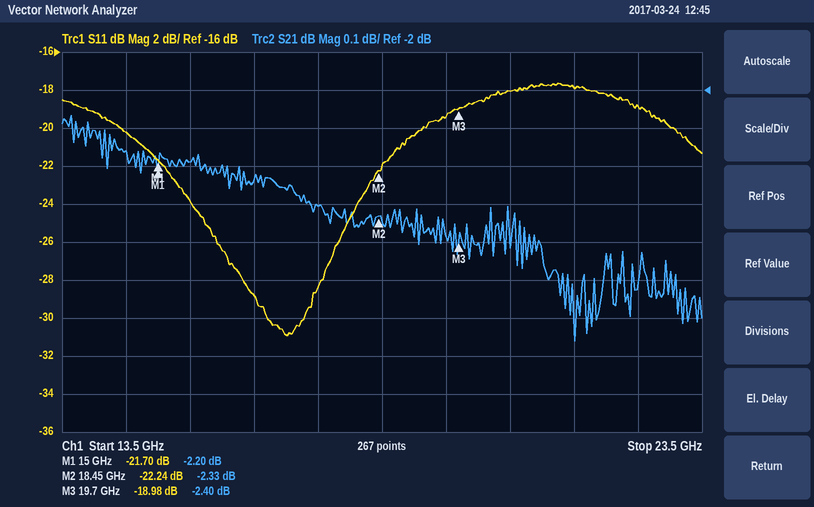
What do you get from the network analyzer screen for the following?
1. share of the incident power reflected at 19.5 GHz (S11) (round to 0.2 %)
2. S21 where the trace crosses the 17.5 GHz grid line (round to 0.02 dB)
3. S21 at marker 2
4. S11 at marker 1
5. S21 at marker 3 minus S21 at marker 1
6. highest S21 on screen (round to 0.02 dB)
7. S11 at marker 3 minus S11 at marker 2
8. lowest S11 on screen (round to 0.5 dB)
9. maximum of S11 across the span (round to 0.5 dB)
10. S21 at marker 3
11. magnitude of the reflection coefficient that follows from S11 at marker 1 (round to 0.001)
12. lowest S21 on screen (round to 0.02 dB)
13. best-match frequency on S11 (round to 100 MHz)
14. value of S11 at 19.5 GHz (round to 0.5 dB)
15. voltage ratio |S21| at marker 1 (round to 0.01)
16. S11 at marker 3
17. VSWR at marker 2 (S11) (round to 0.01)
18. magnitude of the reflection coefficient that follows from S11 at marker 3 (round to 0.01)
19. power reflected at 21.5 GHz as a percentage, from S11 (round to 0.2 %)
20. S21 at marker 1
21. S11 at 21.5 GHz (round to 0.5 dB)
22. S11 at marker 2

1.2 %
-2.30 dB
-2.33 dB
-21.70 dB
-0.20 dB
-2.06 dB
3.26 dB
-31.0 dB
-17.5 dB
-2.40 dB
0.082
-2.66 dB
17.0 GHz
-19.5 dB
0.78
-18.98 dB
1.17
0.11
1.6 %
-2.20 dB
-18.0 dB
-22.24 dB
